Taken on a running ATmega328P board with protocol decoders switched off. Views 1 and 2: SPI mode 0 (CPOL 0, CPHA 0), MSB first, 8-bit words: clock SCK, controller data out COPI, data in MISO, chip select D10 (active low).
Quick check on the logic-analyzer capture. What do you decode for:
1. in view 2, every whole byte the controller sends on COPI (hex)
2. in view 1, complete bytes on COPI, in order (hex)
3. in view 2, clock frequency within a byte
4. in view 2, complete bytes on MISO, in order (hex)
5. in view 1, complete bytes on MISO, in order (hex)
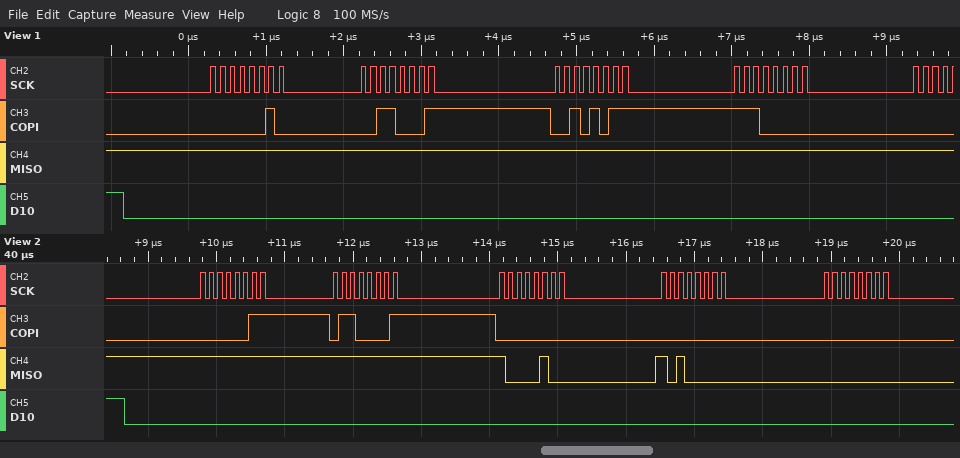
03 61 00 00 00
02 31 2B E0
8 MHz
FF FF 84 A0 00
FF FF FF FF
